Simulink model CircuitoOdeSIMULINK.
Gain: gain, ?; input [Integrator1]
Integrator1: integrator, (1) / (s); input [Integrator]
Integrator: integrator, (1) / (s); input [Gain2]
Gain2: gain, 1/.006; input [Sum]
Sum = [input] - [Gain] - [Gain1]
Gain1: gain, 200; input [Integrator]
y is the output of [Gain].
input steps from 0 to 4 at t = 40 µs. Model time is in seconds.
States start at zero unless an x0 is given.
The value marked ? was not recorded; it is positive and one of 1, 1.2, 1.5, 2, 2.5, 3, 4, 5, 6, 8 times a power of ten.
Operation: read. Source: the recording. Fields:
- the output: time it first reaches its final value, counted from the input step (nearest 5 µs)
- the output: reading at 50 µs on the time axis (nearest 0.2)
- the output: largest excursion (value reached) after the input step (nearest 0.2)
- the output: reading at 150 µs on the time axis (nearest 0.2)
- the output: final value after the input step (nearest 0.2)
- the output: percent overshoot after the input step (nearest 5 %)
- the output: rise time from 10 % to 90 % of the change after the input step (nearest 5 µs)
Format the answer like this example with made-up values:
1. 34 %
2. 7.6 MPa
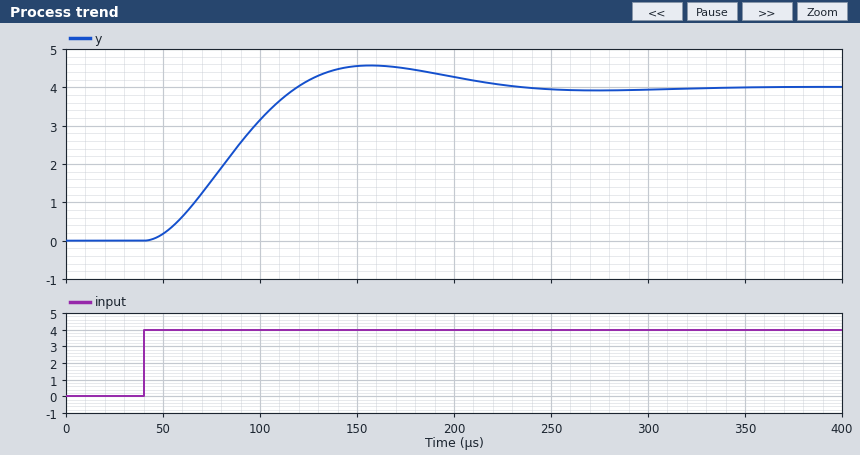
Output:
1. 80 µs
2. 0.2
3. 4.6
4. 4.6
5. 4.0
6. 15 %
7. 55 µs
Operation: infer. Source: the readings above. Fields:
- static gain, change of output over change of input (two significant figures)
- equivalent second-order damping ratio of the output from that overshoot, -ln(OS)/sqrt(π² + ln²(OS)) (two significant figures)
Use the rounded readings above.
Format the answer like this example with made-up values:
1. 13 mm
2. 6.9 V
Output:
1. 1.0
2. 0.52
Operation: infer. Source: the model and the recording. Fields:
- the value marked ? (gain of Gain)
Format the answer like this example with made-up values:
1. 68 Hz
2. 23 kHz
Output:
1. 6e+06
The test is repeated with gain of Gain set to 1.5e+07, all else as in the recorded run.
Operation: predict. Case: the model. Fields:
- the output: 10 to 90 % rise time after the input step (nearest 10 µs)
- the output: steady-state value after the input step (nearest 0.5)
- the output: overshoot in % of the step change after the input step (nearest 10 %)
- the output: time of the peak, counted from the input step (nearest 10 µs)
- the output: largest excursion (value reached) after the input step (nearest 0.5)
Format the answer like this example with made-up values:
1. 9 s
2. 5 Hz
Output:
1. 30 µs
2. 4.0
3. 30 %
4. 70 µs
5. 5.5
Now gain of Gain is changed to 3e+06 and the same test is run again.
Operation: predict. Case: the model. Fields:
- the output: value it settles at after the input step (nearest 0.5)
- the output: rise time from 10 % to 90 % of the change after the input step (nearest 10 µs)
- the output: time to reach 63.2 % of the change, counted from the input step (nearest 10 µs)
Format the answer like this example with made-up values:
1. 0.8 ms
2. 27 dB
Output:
1. 4.0
2. 100 µs
3. 80 µs
